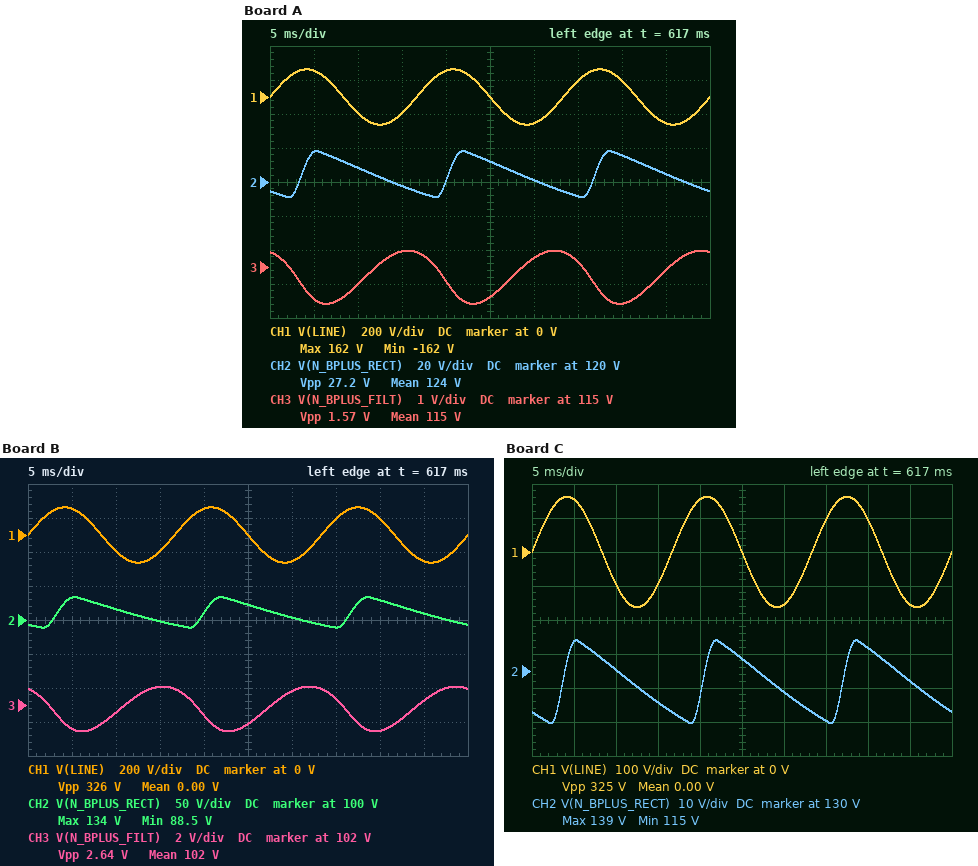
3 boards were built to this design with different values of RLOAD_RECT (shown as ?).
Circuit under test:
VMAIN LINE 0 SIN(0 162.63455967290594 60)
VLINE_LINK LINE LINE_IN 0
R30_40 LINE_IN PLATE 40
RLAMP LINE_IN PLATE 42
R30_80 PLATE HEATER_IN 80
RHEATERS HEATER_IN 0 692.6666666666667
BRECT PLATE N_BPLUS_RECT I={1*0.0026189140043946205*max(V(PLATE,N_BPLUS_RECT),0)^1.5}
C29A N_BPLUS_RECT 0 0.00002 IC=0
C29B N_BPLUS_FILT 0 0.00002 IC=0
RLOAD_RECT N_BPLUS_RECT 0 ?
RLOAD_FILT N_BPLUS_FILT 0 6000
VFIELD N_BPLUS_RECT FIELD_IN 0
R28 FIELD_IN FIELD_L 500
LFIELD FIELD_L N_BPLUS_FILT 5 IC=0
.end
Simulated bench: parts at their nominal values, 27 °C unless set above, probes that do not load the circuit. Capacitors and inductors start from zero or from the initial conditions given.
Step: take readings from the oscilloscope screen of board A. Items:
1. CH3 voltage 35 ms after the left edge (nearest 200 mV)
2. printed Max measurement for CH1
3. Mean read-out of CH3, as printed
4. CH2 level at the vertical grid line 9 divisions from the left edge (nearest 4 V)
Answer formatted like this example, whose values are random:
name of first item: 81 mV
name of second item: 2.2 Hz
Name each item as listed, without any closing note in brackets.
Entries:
CH3 voltage 35 ms after the left edge: 115.2 V
printed Max measurement for CH1: 162 V
Mean read-out of CH3, as printed: 115 V
CH2 level at the vertical grid line 9 divisions from the left edge: 124 V
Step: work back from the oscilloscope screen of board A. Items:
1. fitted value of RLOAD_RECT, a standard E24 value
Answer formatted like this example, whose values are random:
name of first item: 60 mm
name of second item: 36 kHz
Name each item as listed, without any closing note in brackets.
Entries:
fitted value of RLOAD_RECT, a standard E24 value: 6.2 kΩ
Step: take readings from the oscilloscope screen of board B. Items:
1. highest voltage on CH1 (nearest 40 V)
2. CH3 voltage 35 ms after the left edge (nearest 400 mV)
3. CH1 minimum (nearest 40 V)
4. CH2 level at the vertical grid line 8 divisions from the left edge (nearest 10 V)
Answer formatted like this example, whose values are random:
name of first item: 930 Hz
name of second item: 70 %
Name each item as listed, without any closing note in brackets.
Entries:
highest voltage on CH1: 160 V
CH3 voltage 35 ms after the left edge: 102.4 V
CH1 minimum: -160 V
CH2 level at the vertical grid line 8 divisions from the left edge: 130 V
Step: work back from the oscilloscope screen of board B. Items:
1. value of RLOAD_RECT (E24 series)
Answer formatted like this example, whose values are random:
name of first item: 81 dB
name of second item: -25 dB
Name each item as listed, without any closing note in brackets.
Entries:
value of RLOAD_RECT: 2.2 kΩ
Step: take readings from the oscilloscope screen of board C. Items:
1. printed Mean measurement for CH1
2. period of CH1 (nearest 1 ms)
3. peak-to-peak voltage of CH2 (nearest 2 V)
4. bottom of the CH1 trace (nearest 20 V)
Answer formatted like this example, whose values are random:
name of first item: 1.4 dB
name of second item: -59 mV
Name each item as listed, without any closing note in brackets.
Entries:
printed Mean measurement for CH1: 0.00 V
period of CH1: 17 ms
peak-to-peak voltage of CH2: 24 V
bottom of the CH1 trace: -160 V
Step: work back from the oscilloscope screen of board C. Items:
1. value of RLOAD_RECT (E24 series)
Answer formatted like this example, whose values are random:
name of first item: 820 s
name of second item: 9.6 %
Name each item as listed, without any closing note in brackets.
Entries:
value of RLOAD_RECT: 8.2 kΩ
